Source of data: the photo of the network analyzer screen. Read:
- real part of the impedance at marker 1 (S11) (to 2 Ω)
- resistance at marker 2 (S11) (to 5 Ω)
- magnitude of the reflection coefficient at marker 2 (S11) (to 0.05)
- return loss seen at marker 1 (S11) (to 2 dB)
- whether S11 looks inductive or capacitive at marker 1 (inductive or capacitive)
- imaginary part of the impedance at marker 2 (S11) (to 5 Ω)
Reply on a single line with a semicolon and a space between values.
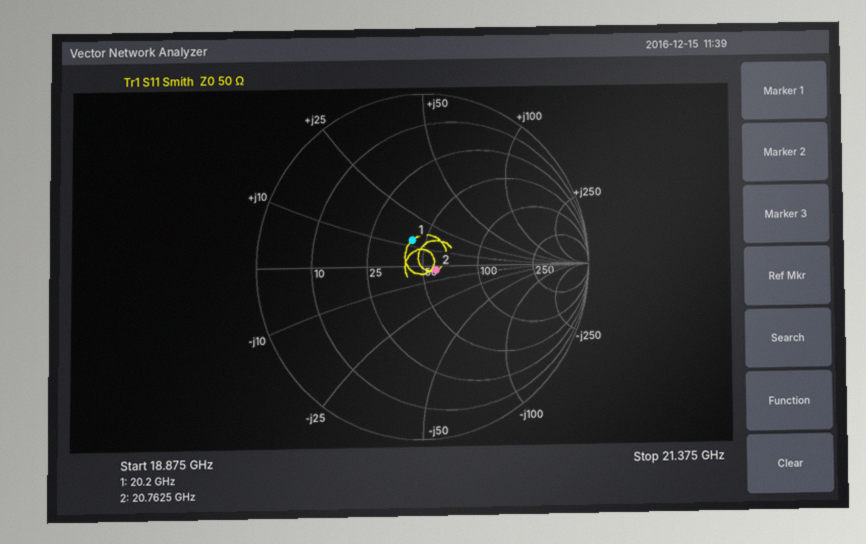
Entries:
42 Ω; 60 Ω; 0.10; 16 dB; inductive; -5 Ω
